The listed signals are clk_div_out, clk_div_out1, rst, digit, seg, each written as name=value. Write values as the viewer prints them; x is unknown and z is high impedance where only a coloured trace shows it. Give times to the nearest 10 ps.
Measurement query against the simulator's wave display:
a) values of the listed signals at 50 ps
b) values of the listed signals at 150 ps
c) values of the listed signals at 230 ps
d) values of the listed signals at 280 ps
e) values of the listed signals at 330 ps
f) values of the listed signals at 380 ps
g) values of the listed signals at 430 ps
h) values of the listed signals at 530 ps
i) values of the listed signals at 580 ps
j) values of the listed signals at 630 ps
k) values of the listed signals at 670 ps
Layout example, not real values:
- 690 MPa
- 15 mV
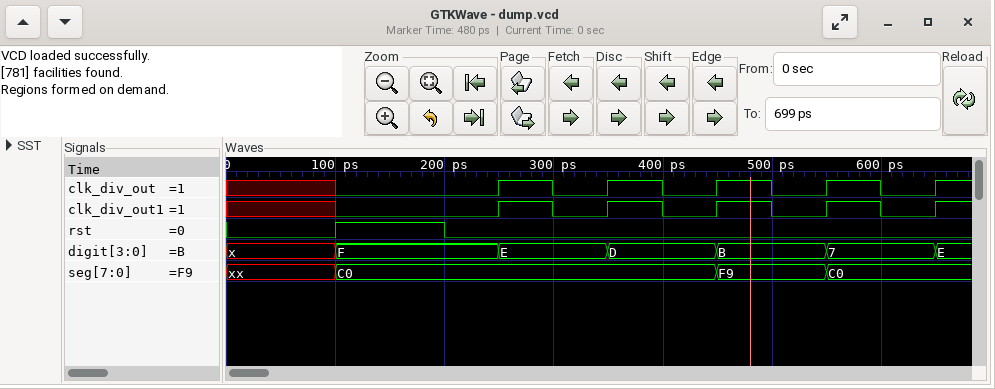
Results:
- clk_div_out=x, clk_div_out1=x, rst=0, digit=x, seg=xx
- clk_div_out=0, clk_div_out1=0, rst=1, digit=F, seg=C0
- clk_div_out=0, clk_div_out1=0, rst=0, digit=F, seg=C0
- clk_div_out=1, clk_div_out1=1, rst=0, digit=E, seg=C0
- clk_div_out=0, clk_div_out1=0, rst=0, digit=E, seg=C0
- clk_div_out=1, clk_div_out1=1, rst=0, digit=D, seg=C0
- clk_div_out=0, clk_div_out1=0, rst=0, digit=D, seg=C0
- clk_div_out=0, clk_div_out1=0, rst=0, digit=B, seg=F9
- clk_div_out=1, clk_div_out1=1, rst=0, digit=7, seg=C0
- clk_div_out=0, clk_div_out1=0, rst=0, digit=7, seg=C0
- clk_div_out=1, clk_div_out1=1, rst=0, digit=E, seg=C0
